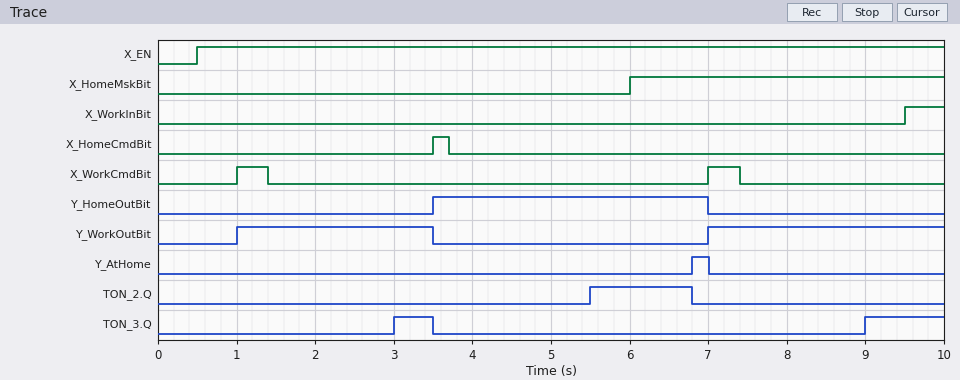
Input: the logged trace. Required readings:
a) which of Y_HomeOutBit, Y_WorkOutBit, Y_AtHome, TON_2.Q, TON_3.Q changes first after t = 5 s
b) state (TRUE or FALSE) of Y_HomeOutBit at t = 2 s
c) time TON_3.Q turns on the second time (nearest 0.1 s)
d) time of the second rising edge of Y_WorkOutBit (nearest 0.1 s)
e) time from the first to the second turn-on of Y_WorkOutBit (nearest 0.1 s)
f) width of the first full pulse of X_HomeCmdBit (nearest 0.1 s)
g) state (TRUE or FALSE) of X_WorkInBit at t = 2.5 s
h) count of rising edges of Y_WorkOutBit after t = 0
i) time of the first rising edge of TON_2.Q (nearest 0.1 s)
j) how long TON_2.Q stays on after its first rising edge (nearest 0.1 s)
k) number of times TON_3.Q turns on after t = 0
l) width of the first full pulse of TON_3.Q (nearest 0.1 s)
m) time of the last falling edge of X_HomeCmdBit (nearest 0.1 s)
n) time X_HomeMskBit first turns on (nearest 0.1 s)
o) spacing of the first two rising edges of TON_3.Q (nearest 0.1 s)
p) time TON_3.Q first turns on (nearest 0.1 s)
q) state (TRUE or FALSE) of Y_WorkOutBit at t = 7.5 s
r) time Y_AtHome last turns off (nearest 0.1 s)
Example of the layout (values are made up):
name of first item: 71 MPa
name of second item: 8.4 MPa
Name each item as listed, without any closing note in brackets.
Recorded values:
which of Y_HomeOutBit, Y_WorkOutBit, Y_AtHome, TON_2.Q, TON_3.Q changes first after t = 5 s: TON_2.Q
state (TRUE or FALSE) of Y_HomeOutBit at t = 2 s: FALSE
time TON_3.Q turns on the second time: 9.0 s
time of the second rising edge of Y_WorkOutBit: 7.0 s
time from the first to the second turn-on of Y_WorkOutBit: 6.0 s
width of the first full pulse of X_HomeCmdBit: 0.2 s
state (TRUE or FALSE) of X_WorkInBit at t = 2.5 s: FALSE
count of rising edges of Y_WorkOutBit after t = 0: 2
time of the first rising edge of TON_2.Q: 5.5 s
how long TON_2.Q stays on after its first rising edge: 1.3 s
number of times TON_3.Q turns on after t = 0: 2
width of the first full pulse of TON_3.Q: 0.5 s
time of the last falling edge of X_HomeCmdBit: 3.7 s
time X_HomeMskBit first turns on: 6.0 s
spacing of the first two rising edges of TON_3.Q: 6.0 s
time TON_3.Q first turns on: 3.0 s
state (TRUE or FALSE) of Y_WorkOutBit at t = 7.5 s: TRUE
time Y_AtHome last turns off: 7.0 s
